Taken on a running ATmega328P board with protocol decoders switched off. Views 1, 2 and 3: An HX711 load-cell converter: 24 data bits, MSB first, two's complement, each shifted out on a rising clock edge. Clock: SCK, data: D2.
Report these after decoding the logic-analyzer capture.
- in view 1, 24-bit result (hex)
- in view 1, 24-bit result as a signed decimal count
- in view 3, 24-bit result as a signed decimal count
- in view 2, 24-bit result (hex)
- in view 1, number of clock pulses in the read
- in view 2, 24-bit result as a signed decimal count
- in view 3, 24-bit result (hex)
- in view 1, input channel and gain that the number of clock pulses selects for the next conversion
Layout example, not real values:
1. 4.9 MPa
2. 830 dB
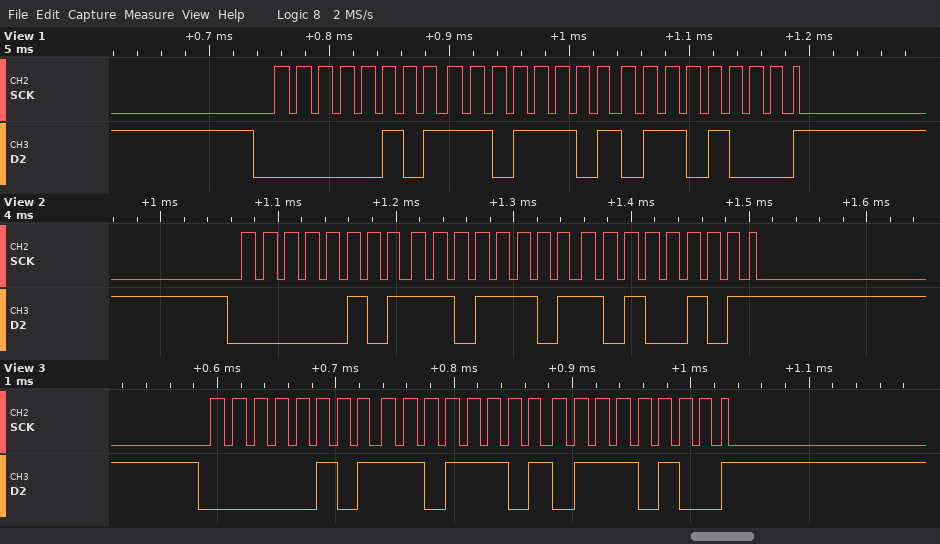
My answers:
1. 0x05DD68
2. 384360
3. 384372
4. 0x05DDA5
5. 25
6. 384421
7. 0x05DD74
8. channel A, gain 128
